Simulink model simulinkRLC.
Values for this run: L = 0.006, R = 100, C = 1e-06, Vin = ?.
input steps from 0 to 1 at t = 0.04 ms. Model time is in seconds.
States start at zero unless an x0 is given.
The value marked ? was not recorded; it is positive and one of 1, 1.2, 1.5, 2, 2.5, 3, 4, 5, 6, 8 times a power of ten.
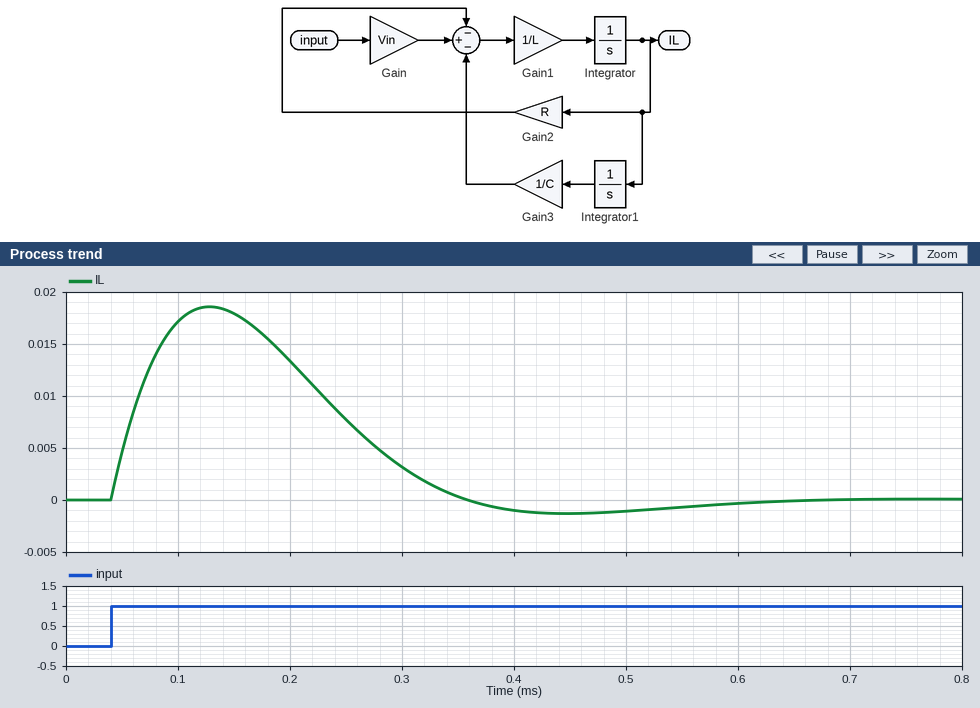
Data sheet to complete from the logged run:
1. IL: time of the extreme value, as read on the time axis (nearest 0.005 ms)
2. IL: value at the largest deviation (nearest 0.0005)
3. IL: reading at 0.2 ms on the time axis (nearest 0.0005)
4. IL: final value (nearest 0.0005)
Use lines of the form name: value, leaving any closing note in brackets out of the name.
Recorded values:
IL: time of the extreme value, as read on the time axis: 0.130 ms
IL: value at the largest deviation: 0.0185
IL: reading at 0.2 ms on the time axis: 0.0135
IL: final value: 0.0000
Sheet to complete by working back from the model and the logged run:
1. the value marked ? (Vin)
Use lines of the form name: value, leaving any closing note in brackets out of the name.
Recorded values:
the value marked ?: 3
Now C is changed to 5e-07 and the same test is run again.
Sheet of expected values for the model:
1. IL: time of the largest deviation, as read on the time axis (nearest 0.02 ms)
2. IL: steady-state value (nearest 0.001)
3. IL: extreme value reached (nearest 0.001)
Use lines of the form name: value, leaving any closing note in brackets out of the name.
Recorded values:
IL: time of the largest deviation, as read on the time axis: 0.10 ms
IL: steady-state value: 0.000
IL: extreme value reached: 0.016
